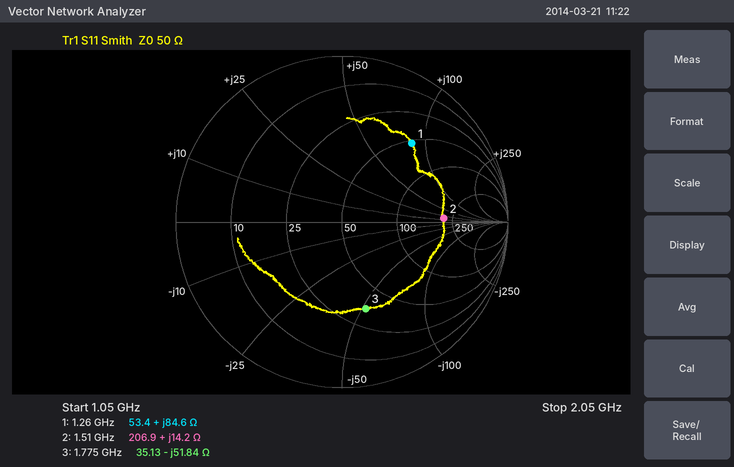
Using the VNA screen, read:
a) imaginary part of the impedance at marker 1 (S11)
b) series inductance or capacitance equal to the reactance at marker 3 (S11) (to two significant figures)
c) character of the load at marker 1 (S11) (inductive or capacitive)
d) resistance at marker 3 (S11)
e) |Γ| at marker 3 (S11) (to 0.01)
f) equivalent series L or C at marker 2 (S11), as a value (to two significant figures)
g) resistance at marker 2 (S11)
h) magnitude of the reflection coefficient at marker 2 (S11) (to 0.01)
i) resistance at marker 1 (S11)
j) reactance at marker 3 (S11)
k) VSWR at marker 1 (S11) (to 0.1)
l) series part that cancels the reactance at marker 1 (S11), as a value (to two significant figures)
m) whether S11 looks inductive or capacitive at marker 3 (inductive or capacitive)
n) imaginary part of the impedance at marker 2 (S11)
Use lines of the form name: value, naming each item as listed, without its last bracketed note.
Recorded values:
imaginary part of the impedance at marker 1: +84.6 Ω
series inductance or capacitance equal to the reactance at marker 3 (S11): 1.7 pF
character of the load at marker 1 (S11): inductive
resistance at marker 3: 35.13 Ω
|Γ| at marker 3 (S11): 0.54
equivalent series L or C at marker 2 (S11), as a value: 1.5 nH
resistance at marker 2: 206.9 Ω
magnitude of the reflection coefficient at marker 2 (S11): 0.61
resistance at marker 1: 53.4 Ω
reactance at marker 3: -51.84 Ω
VSWR at marker 1 (S11): 4.5
series part that cancels the reactance at marker 1 (S11), as a value: 1.5 pF
whether S11 looks inductive or capacitive at marker 3: capacitive
imaginary part of the impedance at marker 2: +14.2 Ω
